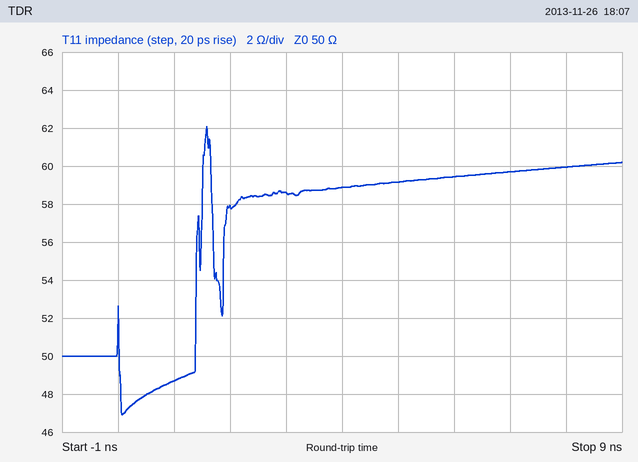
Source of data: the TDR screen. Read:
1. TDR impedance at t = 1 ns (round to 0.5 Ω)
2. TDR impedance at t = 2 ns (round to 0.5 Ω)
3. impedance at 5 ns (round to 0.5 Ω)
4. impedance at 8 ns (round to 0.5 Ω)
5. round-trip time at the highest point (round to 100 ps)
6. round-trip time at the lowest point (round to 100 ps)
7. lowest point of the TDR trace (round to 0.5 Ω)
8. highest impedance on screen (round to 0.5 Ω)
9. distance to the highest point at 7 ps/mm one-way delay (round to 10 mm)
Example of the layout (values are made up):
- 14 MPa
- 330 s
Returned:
- 48.5 Ω
- 58.0 Ω
- 59.0 Ω
- 60.0 Ω
- 1.6 ns
- 100 ps
- 47.0 Ω
- 62.0 Ω
- 110 mm
